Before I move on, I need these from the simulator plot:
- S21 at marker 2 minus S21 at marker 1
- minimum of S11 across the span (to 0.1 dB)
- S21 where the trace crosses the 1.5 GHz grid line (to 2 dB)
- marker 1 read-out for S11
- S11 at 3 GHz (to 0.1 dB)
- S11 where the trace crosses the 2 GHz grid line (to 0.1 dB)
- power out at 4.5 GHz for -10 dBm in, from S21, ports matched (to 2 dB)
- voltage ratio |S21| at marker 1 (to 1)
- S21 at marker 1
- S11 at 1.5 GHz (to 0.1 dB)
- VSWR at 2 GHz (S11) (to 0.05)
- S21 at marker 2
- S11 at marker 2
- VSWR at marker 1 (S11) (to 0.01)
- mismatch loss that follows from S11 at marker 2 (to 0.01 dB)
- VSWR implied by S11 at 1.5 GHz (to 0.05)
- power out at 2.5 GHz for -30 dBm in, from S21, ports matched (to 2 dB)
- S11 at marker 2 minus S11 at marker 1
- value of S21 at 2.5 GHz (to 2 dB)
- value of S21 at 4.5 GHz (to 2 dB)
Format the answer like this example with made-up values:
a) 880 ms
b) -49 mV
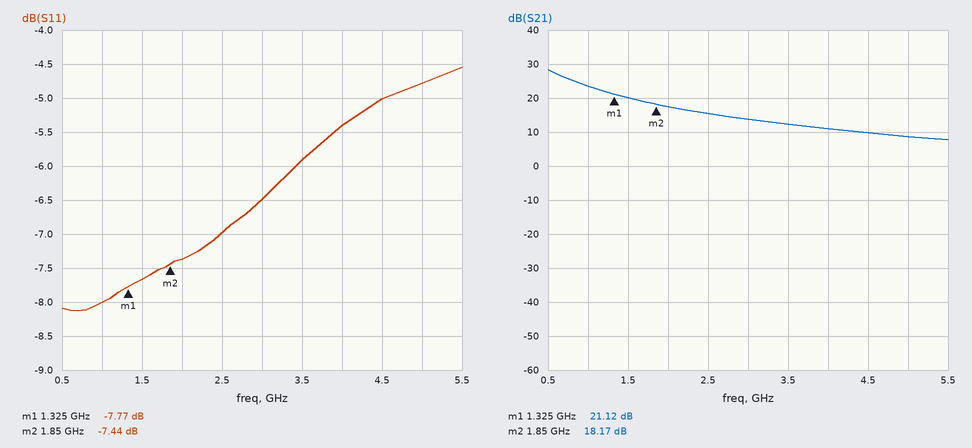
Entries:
a) -2.95 dB
b) -8.1 dB
c) 20 dB
d) -7.77 dB
e) -6.5 dB
f) -7.4 dB
g) 0 dBm
h) 11
i) 21.12 dB
j) -7.7 dB
k) 2.50
l) 18.17 dB
m) -7.44 dB
n) 2.38
o) 0.86 dB
p) 2.40
q) -14 dBm
r) 0.33 dB
s) 16 dB
t) 10 dB
